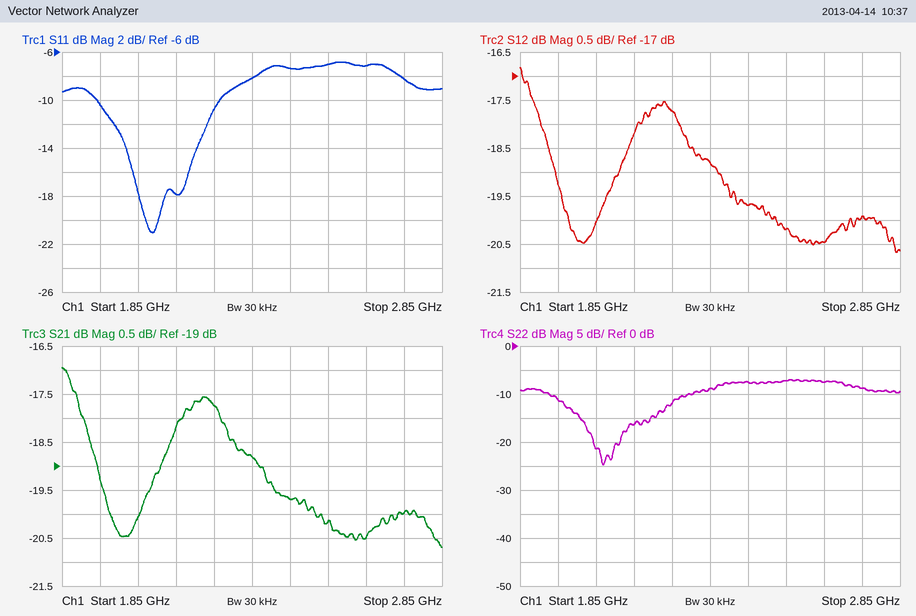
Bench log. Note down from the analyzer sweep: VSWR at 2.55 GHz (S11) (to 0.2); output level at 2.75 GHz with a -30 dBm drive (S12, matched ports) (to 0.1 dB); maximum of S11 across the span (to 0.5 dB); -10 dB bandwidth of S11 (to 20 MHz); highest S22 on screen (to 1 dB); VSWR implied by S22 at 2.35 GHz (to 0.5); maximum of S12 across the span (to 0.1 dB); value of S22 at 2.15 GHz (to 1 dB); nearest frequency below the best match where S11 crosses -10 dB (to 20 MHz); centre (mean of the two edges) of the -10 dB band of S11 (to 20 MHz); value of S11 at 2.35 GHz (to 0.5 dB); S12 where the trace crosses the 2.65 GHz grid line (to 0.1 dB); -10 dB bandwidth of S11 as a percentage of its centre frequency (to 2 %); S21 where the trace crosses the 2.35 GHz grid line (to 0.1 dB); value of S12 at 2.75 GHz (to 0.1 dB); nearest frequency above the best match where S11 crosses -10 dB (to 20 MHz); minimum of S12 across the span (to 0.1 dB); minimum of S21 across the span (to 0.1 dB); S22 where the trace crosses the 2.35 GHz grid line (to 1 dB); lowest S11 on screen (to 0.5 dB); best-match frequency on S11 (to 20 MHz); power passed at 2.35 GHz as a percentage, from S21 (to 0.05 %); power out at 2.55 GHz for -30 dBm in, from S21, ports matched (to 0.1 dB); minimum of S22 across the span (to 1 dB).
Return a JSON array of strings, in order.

["2.6", "-49.9 dBm", "-7.0 dB", "320 MHz", "-7 dB", "2.0", "-16.8 dB", "-16 dB", "1.94 GHz", "2.10 GHz", "-8.0 dB", "-20.5 dB", "16 %", "-18.8 dB", "-19.9 dB", "2.26 GHz", "-20.7 dB", "-20.7 dB", "-9 dB", "-21.0 dB", "2.08 GHz", "1.30 %", "-50.2 dBm", "-25 dB"]
